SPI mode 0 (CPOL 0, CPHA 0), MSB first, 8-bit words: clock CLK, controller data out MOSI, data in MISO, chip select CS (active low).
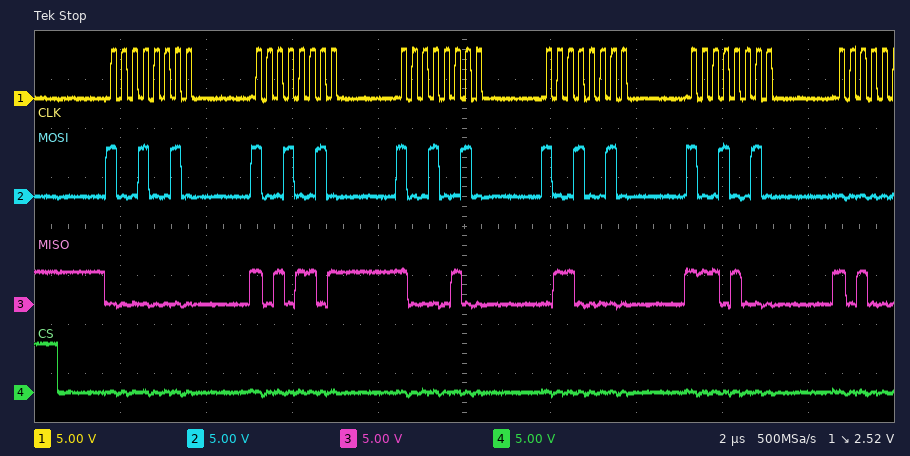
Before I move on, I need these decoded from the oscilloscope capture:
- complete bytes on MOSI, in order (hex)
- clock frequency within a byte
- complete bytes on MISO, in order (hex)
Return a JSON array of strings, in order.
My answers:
["92 92 92 92 92", "4 MHz", "00 AD 84 60 E8"]
